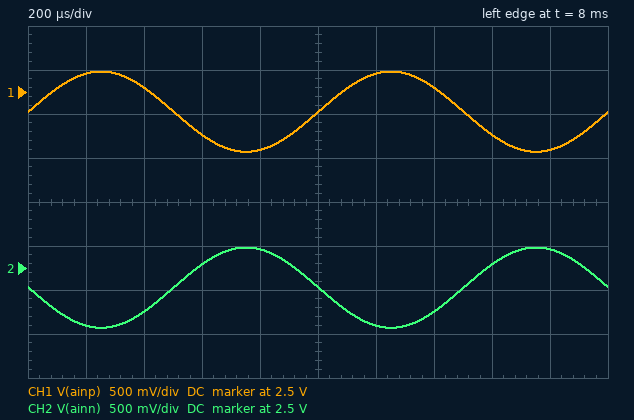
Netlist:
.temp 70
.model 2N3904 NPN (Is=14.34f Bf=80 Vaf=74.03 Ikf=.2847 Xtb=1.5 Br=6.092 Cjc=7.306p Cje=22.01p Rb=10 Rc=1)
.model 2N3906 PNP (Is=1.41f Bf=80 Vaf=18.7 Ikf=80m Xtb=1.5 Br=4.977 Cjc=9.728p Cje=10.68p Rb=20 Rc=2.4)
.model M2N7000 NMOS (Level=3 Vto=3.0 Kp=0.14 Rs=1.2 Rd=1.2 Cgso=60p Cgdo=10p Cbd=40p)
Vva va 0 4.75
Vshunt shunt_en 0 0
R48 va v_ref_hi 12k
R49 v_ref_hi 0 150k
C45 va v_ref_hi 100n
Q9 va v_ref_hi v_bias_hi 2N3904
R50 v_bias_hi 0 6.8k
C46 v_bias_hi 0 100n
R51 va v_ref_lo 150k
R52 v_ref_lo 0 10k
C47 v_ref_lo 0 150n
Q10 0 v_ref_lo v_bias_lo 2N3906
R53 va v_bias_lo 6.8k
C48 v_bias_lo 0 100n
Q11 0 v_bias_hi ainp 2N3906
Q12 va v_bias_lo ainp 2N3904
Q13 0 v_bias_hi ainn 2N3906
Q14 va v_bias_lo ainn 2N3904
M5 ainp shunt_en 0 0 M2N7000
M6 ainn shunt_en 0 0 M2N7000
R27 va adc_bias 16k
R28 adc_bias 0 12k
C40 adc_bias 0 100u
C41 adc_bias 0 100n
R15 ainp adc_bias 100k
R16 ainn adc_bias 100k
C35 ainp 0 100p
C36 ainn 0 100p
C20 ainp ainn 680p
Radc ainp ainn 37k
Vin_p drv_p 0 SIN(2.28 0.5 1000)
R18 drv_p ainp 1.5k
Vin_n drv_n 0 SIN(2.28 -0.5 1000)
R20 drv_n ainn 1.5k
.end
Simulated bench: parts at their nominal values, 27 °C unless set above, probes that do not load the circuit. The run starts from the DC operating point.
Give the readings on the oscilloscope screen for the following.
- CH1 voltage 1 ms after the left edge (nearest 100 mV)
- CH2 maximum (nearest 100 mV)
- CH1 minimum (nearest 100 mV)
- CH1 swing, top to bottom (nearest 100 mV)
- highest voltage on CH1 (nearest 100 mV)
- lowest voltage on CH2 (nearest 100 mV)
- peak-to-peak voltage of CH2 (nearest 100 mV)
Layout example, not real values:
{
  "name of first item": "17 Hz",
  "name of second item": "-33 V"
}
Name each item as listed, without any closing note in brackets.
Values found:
{
  "CH1 voltage 1 ms after the left edge": "2.3 V",
  "CH2 maximum": "2.7 V",
  "CH1 minimum": "1.8 V",
  "CH1 swing, top to bottom": "900 mV",
  "highest voltage on CH1": "2.7 V",
  "lowest voltage on CH2": "1.8 V",
  "peak-to-peak voltage of CH2": "900 mV"
}
